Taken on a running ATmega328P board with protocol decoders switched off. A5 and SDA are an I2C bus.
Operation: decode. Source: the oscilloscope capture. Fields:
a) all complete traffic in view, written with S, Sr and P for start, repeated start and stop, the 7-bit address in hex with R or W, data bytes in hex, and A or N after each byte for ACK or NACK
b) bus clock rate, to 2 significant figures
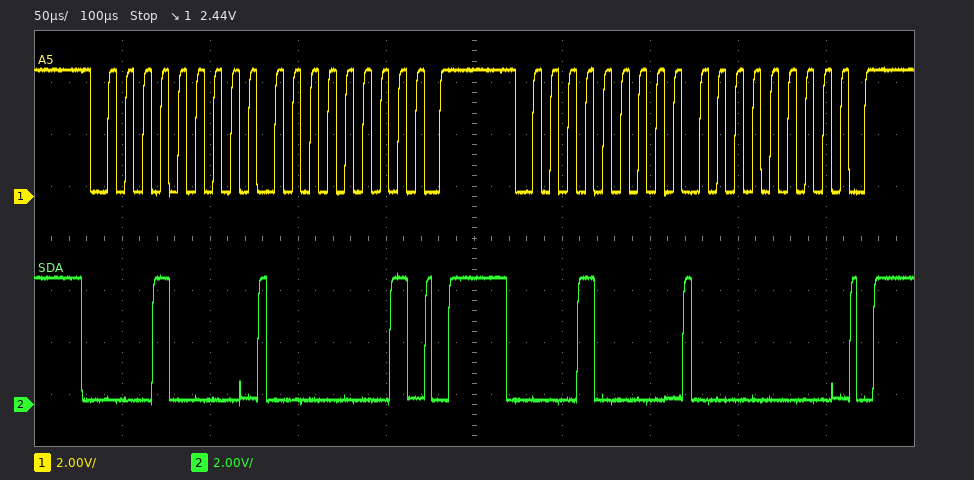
S 08W A 01 A P S 08W A 00 A P
100 kHz
